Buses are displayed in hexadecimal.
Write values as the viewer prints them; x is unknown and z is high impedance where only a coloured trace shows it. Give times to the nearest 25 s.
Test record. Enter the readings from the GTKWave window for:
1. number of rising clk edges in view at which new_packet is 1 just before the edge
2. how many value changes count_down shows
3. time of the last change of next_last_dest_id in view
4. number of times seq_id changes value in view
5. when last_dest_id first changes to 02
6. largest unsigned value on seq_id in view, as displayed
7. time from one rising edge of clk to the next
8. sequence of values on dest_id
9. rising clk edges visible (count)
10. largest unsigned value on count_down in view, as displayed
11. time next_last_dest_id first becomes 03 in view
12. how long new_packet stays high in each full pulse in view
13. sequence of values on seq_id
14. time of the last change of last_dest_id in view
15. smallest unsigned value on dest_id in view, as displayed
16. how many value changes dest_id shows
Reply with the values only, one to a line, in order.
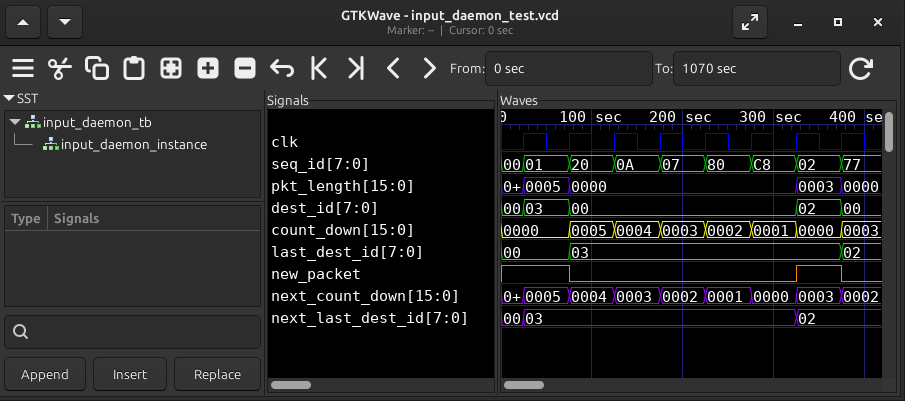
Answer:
3
7
325 s
8
375 s
C8
50 s
00, 03, 00, 02, 00
8
0005
25 s
50 s
00, 01, 20, 0A, 07, 80, C8, 02, 77
375 s
00
4
